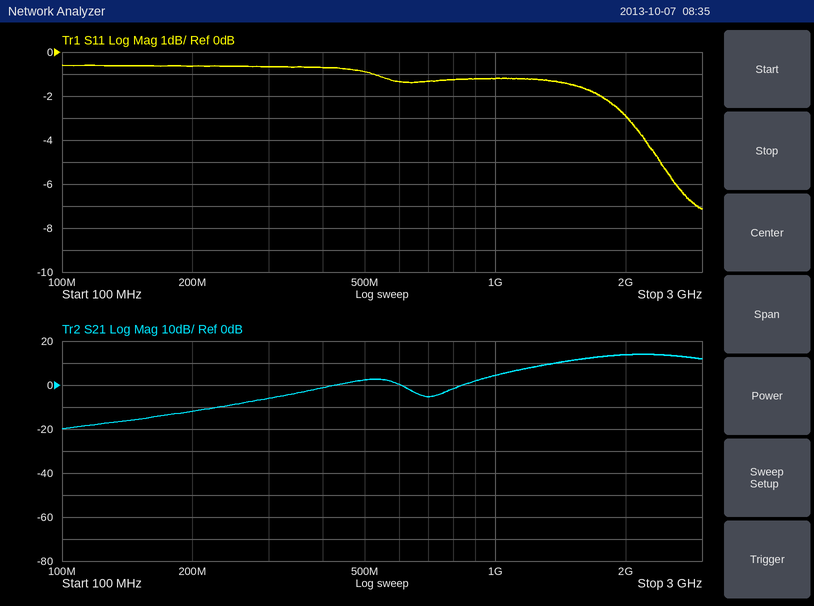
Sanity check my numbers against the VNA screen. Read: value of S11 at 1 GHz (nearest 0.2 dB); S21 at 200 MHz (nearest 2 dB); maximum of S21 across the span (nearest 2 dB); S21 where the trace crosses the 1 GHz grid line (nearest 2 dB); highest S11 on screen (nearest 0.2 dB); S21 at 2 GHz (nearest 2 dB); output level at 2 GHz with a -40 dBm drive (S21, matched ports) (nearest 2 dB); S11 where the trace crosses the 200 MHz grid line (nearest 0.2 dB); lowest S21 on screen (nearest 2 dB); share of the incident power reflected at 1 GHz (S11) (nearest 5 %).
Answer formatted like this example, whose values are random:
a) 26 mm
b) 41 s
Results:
a) -1.2 dB
b) -12 dB
c) 14 dB
d) 4 dB
e) -0.6 dB
f) 14 dB
g) -26 dBm
h) -0.6 dB
i) -20 dB
j) 75 %
